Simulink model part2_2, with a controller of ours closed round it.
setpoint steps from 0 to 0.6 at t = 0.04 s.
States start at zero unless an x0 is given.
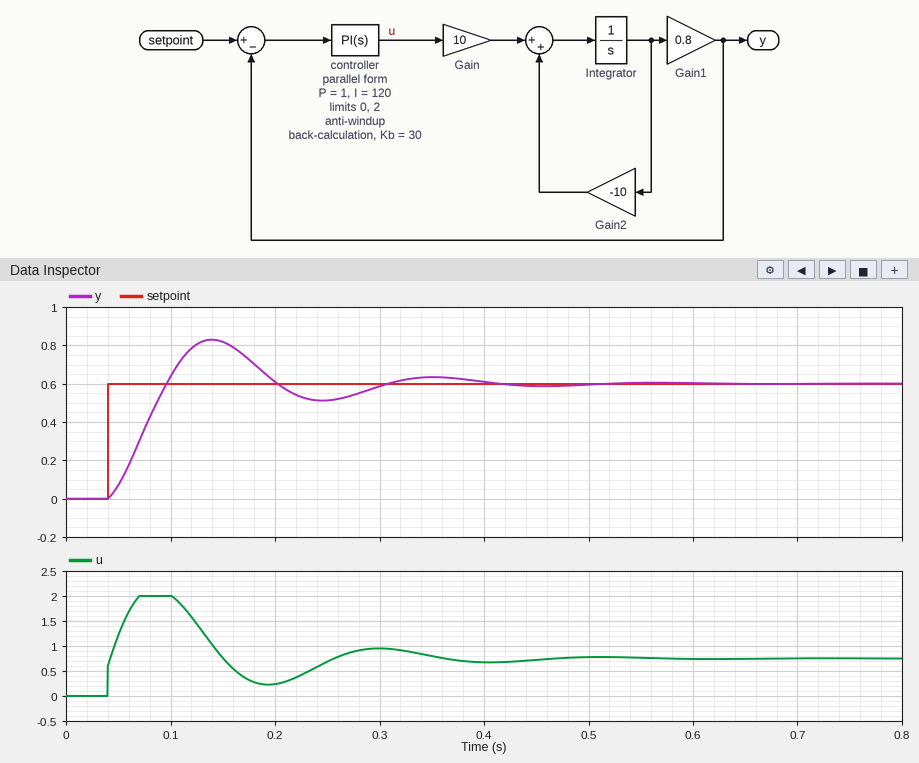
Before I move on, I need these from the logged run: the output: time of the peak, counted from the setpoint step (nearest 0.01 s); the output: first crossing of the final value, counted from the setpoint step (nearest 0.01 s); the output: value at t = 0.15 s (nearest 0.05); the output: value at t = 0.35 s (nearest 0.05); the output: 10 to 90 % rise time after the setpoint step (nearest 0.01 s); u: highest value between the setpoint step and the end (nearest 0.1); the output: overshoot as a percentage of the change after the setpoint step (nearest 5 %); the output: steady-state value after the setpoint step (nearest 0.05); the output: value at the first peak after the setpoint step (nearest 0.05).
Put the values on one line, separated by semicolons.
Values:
0.10 s; 0.06 s; 0.80; 0.65; 0.04 s; 2.0; 40 %; 0.60; 0.85
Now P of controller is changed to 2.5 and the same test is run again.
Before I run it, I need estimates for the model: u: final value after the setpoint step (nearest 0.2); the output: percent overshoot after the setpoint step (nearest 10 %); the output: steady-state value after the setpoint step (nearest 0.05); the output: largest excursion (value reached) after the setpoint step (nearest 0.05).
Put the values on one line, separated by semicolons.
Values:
0.8; 20 %; 0.60; 0.75
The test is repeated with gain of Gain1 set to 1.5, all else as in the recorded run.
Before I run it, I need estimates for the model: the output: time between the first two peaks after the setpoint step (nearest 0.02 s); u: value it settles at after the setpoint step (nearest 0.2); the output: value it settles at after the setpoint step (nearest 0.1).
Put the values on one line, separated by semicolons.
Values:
0.16 s; 0.4; 0.6
